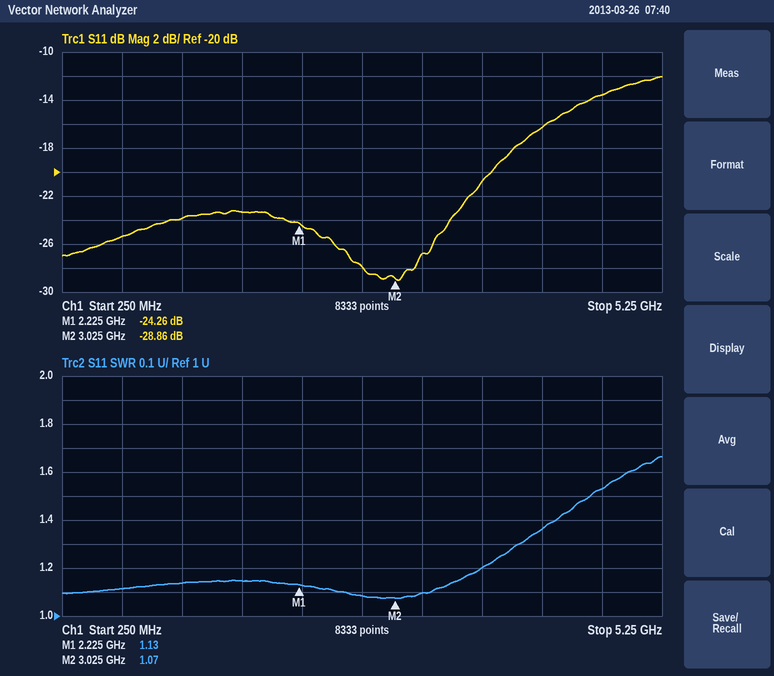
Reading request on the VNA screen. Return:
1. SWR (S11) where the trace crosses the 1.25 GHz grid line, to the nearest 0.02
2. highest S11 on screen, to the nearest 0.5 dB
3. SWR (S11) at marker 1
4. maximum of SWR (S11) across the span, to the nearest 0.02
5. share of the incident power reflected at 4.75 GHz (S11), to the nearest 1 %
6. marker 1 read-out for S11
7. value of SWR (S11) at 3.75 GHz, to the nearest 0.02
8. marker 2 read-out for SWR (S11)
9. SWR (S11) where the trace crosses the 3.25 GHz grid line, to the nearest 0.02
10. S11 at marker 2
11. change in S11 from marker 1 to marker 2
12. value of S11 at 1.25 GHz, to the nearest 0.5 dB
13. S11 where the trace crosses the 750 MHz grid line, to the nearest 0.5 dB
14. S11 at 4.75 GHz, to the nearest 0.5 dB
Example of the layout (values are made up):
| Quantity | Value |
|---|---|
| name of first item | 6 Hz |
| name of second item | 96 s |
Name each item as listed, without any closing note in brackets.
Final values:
| Quantity | Value |
|---|---|
| SWR (S11) where the trace crosses the 1.25 GHz grid line, to the nearest 0.02 | 1.14 |
| highest S11 on screen, to the nearest 0.5 dB | -12.0 dB |
| SWR (S11) at marker 1 | 1.13 |
| maximum of SWR (S11) across the span, to the nearest 0.02 | 1.66 |
| share of the incident power reflected at 4.75 GHz (S11), to the nearest 1 % | 4 % |
| marker 1 read-out for S11 | -24.26 dB |
| value of SWR (S11) at 3.75 GHz, to the nearest 0.02 | 1.20 |
| marker 2 read-out for SWR | 1.07 |
| SWR (S11) where the trace crosses the 3.25 GHz grid line, to the nearest 0.02 | 1.10 |
| S11 at marker 2 | -28.86 dB |
| change in S11 from marker 1 to marker 2 | -4.60 dB |
| value of S11 at 1.25 GHz, to the nearest 0.5 dB | -24.0 dB |
| S11 where the trace crosses the 750 MHz grid line, to the nearest 0.5 dB | -25.5 dB |
| S11 at 4.75 GHz, to the nearest 0.5 dB | -13.5 dB |
